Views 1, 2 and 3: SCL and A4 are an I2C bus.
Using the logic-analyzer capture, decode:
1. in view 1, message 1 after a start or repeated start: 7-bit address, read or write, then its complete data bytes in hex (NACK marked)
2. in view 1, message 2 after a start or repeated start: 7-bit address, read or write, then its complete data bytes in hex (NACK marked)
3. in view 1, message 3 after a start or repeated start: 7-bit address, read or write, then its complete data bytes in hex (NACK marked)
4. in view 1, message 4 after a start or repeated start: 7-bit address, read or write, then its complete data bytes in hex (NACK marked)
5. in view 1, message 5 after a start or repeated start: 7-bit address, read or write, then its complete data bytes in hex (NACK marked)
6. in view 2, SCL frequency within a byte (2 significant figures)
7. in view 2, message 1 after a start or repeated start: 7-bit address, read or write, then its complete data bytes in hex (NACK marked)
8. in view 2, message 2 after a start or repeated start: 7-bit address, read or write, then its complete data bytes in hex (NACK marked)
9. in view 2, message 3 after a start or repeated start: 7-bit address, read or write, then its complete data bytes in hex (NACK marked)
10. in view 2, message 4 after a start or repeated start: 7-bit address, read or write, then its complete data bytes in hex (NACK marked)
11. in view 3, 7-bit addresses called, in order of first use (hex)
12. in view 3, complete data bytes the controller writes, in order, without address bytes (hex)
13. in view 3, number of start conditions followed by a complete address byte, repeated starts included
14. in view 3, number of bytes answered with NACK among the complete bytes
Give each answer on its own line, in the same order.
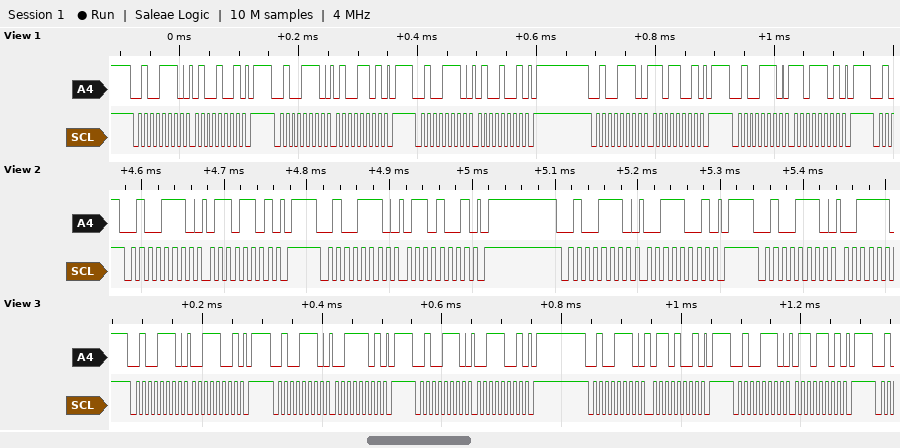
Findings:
0x27 write: 49
0x27 write: 4D
0x27 write: 49
0x27 write: D9
0x27 write: DD
100 kHz
0x27 write: 6D
0x27 write: 69
0x27 write: 39
0x27 write
0x27
39 3D 39 69 6D
5
0
